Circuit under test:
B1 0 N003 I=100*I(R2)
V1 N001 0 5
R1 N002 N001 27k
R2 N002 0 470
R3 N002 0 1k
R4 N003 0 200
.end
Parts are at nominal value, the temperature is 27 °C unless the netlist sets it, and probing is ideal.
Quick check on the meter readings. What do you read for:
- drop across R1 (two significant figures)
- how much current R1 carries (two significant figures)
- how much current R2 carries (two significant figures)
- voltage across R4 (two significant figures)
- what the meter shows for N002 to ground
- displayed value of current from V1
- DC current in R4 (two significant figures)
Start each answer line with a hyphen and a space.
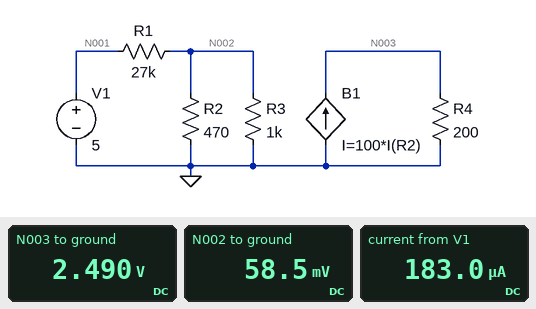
- 4.9 V
- 180 µA
- 120 µA
- 2.5 V
- 58.5 mV
- 183.0 µA
- 12 mA
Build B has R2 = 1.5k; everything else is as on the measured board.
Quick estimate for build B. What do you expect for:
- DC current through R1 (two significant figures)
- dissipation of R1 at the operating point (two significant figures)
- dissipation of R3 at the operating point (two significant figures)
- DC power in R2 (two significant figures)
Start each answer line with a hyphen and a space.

- 180 µA
- 890 µW
- 12 µW
- 7.9 µW
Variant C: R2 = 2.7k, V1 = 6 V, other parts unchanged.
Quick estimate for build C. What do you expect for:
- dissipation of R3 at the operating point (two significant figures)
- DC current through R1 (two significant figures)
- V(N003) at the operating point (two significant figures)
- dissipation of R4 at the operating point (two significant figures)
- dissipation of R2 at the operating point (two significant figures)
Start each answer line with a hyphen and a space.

- 25 µW
- 220 µA
- 1.2 V
- 6.8 mW
- 9.2 µW
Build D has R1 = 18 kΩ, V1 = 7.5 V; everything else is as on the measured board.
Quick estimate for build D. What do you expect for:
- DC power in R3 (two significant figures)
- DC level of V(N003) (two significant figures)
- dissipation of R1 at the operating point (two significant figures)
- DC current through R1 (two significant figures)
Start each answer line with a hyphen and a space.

- 17 µW
- 5.6 V
- 3.0 mW
- 410 µA
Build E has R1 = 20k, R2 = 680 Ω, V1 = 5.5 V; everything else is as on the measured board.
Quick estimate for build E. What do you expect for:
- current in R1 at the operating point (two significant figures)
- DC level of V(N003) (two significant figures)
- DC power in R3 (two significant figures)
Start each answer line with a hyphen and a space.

- 270 µA
- 3.2 V
- 12 µW
